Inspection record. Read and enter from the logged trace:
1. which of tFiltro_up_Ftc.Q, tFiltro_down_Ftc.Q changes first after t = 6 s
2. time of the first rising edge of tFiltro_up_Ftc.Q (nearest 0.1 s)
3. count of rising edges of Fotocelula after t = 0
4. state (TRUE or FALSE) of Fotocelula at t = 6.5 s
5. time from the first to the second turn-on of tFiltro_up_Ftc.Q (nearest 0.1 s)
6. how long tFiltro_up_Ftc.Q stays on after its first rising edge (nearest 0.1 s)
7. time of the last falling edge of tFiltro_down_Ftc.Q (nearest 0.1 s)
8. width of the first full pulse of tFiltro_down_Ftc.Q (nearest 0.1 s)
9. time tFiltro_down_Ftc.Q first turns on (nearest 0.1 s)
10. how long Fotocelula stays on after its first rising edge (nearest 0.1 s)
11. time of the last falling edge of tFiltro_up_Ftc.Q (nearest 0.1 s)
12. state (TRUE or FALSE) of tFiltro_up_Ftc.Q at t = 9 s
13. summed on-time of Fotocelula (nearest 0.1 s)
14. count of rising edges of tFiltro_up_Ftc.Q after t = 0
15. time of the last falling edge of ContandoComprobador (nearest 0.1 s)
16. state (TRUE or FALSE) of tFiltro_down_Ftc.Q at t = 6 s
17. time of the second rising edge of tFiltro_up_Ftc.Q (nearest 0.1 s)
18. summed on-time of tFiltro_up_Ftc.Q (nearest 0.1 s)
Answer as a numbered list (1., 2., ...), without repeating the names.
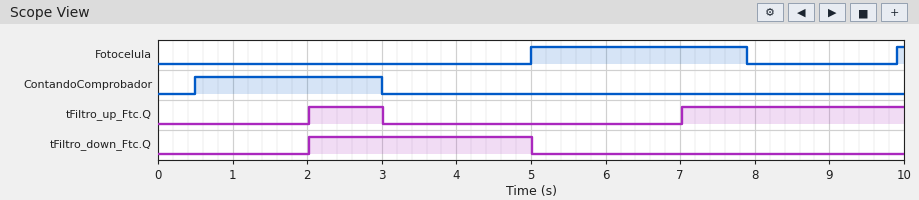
1. tFiltro_up_Ftc.Q
2. 2.0 s
3. 2
4. TRUE
5. 5.0 s
6. 1.0 s
7. 5.0 s
8. 3.0 s
9. 2.0 s
10. 2.9 s
11. 3.0 s
12. TRUE
13. 3.0 s
14. 2
15. 3.0 s
16. FALSE
17. 7.0 s
18. 4.0 s
